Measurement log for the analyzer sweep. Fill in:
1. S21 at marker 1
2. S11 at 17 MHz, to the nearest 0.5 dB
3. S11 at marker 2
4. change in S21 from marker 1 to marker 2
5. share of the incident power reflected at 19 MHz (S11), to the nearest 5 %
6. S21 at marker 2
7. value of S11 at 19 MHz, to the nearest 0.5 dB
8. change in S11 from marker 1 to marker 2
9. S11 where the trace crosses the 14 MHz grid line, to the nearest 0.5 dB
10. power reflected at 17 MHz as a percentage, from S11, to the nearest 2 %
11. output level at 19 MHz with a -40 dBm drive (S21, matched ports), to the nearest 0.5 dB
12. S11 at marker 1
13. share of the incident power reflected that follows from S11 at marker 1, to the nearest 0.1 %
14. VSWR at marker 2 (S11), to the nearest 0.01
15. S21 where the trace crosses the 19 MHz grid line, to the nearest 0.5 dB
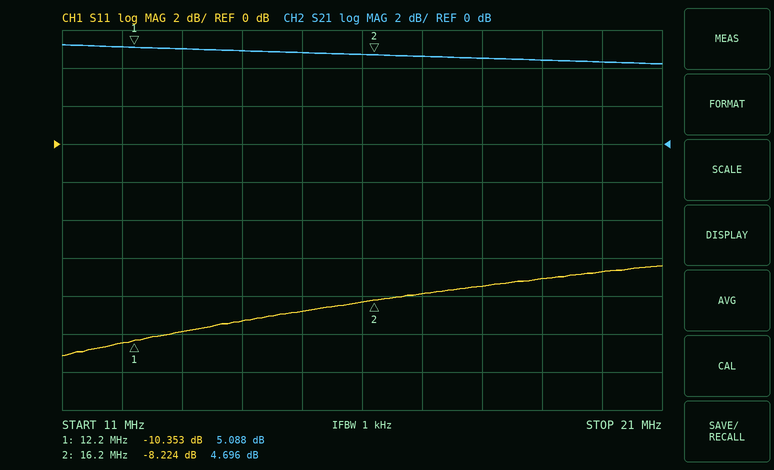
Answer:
5.088 dB
-8.0 dB
-8.224 dB
-0.392 dB
20 %
4.696 dB
-7.0 dB
2.129 dB
-9.5 dB
16 %
-35.5 dBm
-10.353 dB
9.2 %
2.27
4.5 dB
